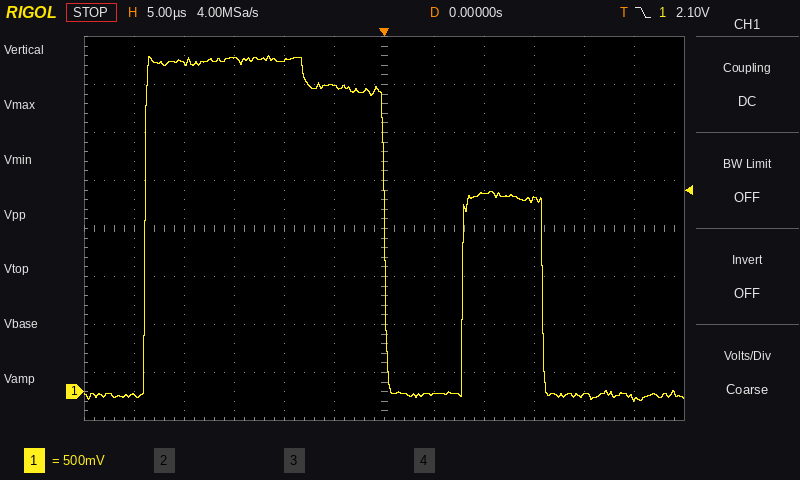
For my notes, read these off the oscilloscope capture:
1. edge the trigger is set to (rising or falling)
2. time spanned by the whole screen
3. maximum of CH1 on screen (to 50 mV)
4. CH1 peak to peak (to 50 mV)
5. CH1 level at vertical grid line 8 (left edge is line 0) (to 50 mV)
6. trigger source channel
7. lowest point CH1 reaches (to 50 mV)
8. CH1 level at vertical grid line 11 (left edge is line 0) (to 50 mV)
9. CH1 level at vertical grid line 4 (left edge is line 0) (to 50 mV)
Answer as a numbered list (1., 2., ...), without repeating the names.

1. falling
2. 60 µs
3. 3.50 V
4. 3.60 V
5. 2.05 V
6. CH1
7. -100 mV
8. -50 mV
9. 3.45 V
